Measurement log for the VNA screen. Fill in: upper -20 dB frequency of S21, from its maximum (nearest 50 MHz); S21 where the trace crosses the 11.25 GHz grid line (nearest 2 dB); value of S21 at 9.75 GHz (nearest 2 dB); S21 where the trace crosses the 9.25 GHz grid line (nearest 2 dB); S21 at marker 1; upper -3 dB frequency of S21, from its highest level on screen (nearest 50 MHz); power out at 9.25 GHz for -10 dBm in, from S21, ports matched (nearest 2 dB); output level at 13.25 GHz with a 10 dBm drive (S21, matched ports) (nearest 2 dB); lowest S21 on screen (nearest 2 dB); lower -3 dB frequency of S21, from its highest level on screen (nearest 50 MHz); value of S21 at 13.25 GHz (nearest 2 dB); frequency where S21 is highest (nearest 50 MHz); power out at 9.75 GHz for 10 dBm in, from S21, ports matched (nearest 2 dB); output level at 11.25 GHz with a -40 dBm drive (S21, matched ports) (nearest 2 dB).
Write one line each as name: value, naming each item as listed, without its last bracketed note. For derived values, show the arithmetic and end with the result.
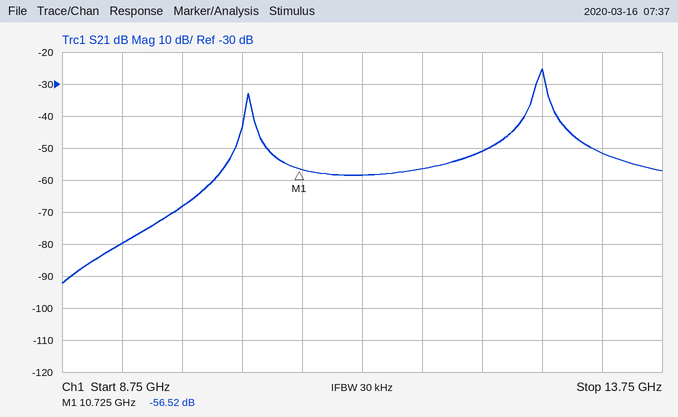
upper -20 dB frequency of S21, from its maximum: 13.00 GHz
S21 where the trace crosses the 11.25 GHz grid line: -58 dB
value of S21 at 9.75 GHz: -68 dB
S21 where the trace crosses the 9.25 GHz grid line: -80 dB
S21 at marker 1: -56.52 dB
upper -3 dB frequency of S21, from its highest level on screen: 12.75 GHz
power out at 9.25 GHz for -10 dBm in, from S21, ports matched: -10 dBm + (-80 dB) = -90 dBm
output level at 13.25 GHz with a 10 dBm drive (S21, matched ports): 10 dBm + (-52 dB) = -42 dBm
lowest S21 on screen: -92 dB
lower -3 dB frequency of S21, from its highest level on screen: 12.70 GHz
value of S21 at 13.25 GHz: -52 dB
frequency where S21 is highest: 12.75 GHz
power out at 9.75 GHz for 10 dBm in, from S21, ports matched: 10 dBm + (-68 dB) = -58 dBm
output level at 11.25 GHz with a -40 dBm drive (S21, matched ports): -40 dBm + (-58 dB) = -98 dBm
